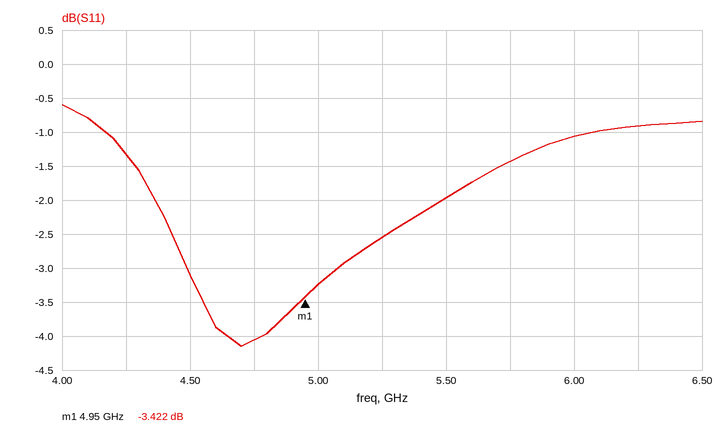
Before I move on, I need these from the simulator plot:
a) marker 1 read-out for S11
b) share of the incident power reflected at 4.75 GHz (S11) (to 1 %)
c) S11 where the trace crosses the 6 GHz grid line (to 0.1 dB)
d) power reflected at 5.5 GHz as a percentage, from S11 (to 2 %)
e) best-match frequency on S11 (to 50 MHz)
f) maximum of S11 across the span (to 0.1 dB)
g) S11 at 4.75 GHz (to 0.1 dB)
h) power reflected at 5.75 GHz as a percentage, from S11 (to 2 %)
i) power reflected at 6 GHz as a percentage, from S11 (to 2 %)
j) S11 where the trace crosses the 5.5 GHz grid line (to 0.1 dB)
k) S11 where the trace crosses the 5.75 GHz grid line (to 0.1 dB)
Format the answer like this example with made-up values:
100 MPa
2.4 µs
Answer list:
-3.422 dB
39 %
-1.1 dB
64 %
4.70 GHz
-0.6 dB
-4.1 dB
72 %
78 %
-2.0 dB
-1.4 dB
